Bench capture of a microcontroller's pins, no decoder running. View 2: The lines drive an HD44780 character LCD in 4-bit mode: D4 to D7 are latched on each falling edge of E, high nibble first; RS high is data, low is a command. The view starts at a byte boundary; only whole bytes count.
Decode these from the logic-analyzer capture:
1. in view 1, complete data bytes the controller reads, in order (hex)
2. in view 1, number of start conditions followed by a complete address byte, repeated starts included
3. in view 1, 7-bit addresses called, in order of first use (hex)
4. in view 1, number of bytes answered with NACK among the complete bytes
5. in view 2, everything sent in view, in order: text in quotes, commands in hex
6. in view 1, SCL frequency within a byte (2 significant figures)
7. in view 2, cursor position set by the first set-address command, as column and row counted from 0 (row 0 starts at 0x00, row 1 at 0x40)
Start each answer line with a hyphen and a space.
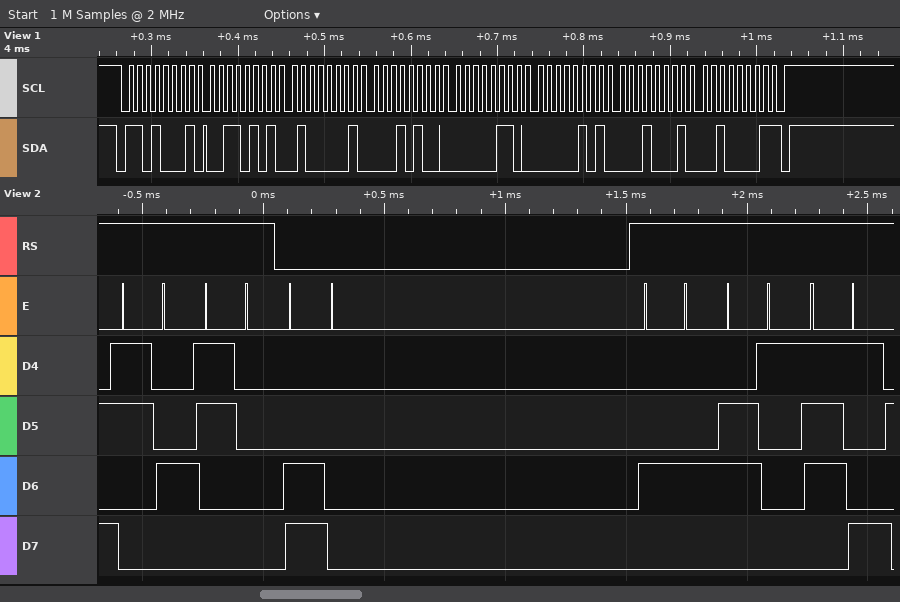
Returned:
- 35 41 14 06 05 11 21
- 1
- 0x68
- 1
- "40" 0xC0 "Day"
- 100 kHz
- column 0, row 1
